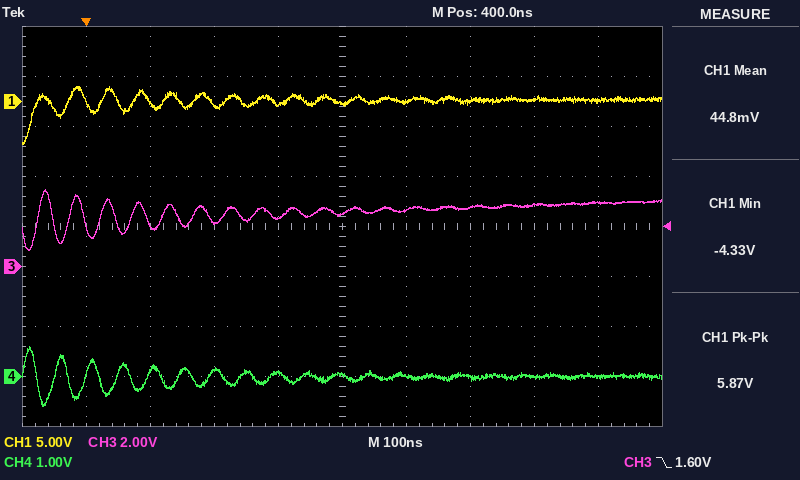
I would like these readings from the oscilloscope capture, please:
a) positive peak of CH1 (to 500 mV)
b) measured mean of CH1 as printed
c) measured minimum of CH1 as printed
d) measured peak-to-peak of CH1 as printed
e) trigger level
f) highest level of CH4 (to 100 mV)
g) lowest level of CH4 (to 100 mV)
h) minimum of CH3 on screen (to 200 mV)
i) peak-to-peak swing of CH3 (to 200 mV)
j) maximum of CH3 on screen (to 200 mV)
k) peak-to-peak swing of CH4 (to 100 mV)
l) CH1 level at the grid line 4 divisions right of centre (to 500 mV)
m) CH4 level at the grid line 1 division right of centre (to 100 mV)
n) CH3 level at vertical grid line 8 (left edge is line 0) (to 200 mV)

1.5 V
44.8 mV
-4.33 V
5.87 V
1.60 V
600 mV
-600 mV
600 mV
2.4 V
3.0 V
1.2 V
0.0 V
0.0 V
2.4 V
